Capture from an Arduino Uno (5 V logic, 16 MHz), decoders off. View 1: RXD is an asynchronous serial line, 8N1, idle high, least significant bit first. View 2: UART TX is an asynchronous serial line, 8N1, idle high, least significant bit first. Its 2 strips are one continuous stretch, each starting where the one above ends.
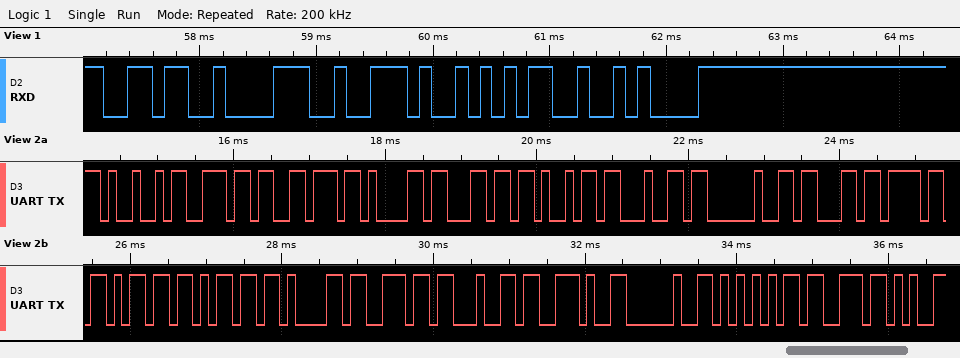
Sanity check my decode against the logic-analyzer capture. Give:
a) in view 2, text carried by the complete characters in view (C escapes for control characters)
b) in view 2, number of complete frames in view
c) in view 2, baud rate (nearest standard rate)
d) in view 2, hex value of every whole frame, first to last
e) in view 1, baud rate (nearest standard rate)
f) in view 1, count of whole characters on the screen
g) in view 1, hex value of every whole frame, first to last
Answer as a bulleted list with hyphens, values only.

- "Invalid command. Us"
- 19
- 9600 baud
- 49 6E 76 61 6C 69 64 20 63 6F 6D 6D 61 6E 64 2E 20 55 73
- 9600 baud
- 5
- 36 38 2E 35 0A
